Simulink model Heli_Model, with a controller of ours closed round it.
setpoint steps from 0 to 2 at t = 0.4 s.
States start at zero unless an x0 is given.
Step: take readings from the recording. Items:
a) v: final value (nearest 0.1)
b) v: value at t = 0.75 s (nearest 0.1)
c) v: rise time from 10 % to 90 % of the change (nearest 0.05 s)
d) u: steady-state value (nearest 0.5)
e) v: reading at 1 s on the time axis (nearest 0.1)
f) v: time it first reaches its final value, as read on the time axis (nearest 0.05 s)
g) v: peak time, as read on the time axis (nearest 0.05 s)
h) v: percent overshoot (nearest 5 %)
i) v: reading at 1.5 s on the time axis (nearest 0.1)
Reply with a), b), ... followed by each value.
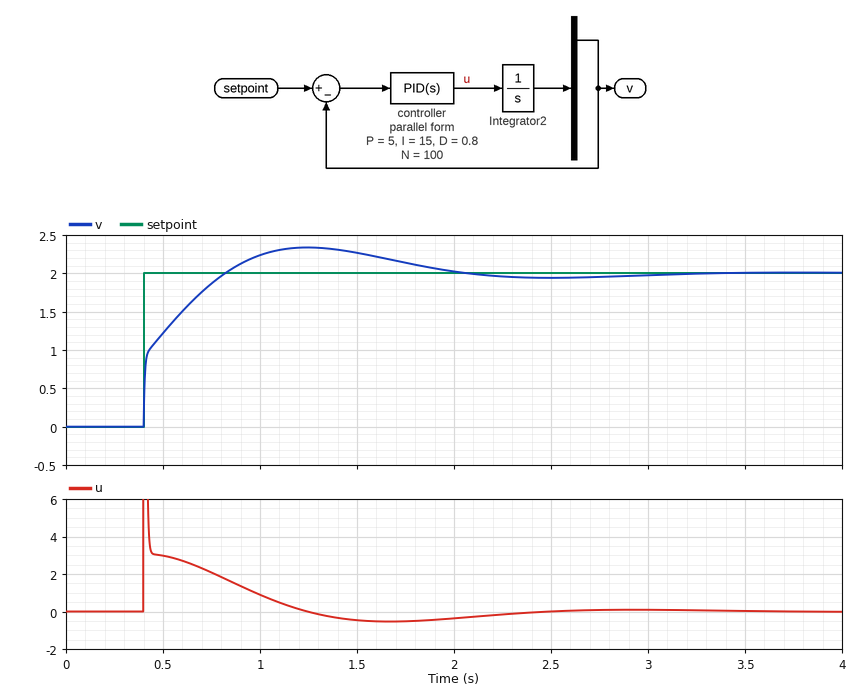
a) 2.0
b) 1.9
c) 0.30 s
d) 0.0
e) 2.2
f) 0.80 s
g) 1.25 s
h) 15 %
i) 2.3
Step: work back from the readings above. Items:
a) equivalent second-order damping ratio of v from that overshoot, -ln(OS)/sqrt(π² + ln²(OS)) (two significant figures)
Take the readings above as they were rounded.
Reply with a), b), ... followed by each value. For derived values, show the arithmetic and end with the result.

a) ln(0.15) = -1.897; 1.897 / sqrt(9.870 + 3.599) = 0.52
